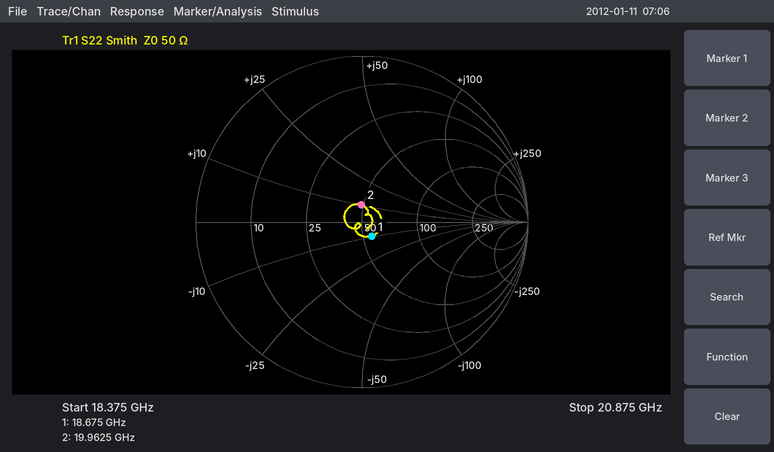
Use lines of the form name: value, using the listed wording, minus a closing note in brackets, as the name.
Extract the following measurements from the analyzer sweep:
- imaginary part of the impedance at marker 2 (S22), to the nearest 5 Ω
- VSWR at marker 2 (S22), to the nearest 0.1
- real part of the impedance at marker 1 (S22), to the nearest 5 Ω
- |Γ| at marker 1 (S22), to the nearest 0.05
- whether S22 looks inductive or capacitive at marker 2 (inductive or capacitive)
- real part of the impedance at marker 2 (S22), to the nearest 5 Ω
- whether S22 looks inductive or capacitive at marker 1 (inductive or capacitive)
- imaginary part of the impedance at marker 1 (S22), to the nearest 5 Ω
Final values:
imaginary part of the impedance at marker 2 (S22), to the nearest 5 Ω: +10 Ω
VSWR at marker 2 (S22), to the nearest 0.1: 1.2
real part of the impedance at marker 1 (S22), to the nearest 5 Ω: 55 Ω
|Γ| at marker 1 (S22), to the nearest 0.05: 0.10
whether S22 looks inductive or capacitive at marker 2: inductive
real part of the impedance at marker 2 (S22), to the nearest 5 Ω: 50 Ω
whether S22 looks inductive or capacitive at marker 1: capacitive
imaginary part of the impedance at marker 1 (S22), to the nearest 5 Ω: -10 Ω
